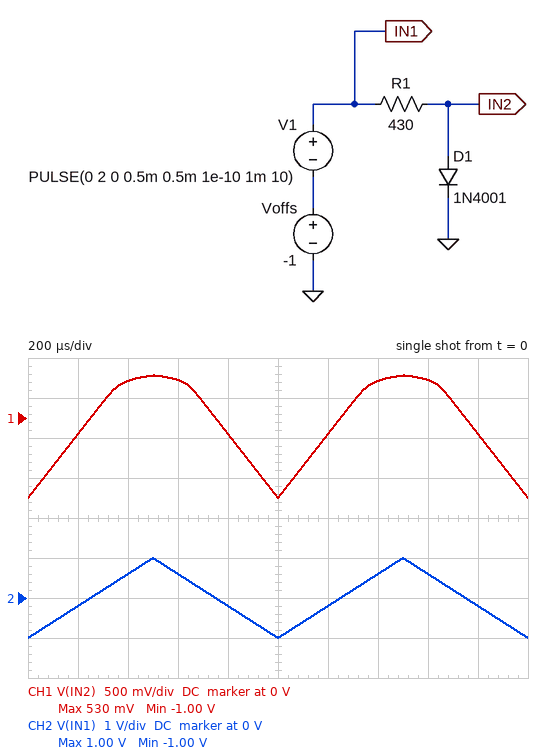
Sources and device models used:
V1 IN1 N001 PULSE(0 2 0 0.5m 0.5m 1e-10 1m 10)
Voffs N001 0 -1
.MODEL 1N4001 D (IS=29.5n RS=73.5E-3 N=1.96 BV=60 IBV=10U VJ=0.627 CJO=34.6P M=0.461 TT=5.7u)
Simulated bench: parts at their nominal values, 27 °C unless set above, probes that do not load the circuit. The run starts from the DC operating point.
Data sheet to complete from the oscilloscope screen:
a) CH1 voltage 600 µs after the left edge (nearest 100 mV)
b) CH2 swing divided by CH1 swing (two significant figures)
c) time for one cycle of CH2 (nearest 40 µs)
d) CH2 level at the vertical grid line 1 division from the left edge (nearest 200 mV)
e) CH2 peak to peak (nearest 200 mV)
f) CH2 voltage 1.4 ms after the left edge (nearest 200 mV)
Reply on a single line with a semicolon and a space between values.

500 mV; 1.3; 1.00 ms; -200 mV; 2.0 V; 600 mV
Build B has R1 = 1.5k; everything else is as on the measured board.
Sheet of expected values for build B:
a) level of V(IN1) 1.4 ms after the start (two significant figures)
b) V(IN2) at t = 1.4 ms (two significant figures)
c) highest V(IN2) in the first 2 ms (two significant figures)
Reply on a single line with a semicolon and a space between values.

600 mV; 420 mV; 470 mV
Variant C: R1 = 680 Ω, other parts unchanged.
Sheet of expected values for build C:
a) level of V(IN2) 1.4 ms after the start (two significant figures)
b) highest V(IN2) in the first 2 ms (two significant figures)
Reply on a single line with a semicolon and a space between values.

450 mV; 510 mV
